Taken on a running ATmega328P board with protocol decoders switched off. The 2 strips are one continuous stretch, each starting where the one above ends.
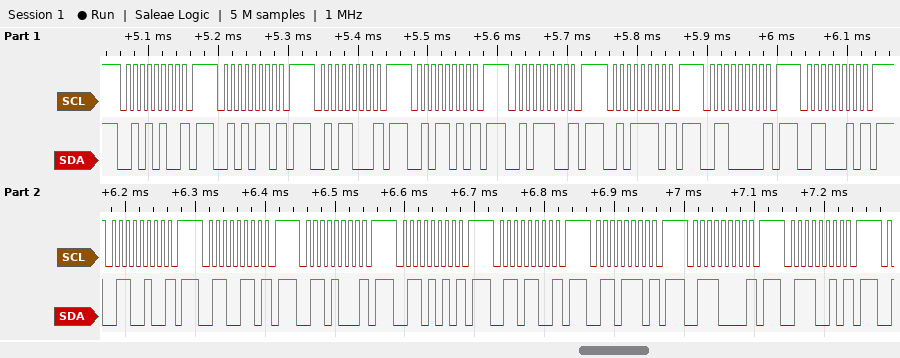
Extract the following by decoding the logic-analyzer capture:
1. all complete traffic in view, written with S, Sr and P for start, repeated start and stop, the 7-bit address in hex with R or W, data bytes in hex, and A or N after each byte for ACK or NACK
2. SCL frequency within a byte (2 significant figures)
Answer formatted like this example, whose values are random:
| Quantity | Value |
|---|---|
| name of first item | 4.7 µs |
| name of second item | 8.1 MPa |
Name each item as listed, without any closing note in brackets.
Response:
| Quantity | Value |
|---|---|
| all complete traffic in view, written with S, Sr and P for start, repeated start and stop, the 7-bit address in hex with R or W, data bytes in hex, and A or N after each byte for ACK or NACK | S 2AW N P S 2BW N P S 2CW N P S 2DW N P S 2EW N P S 2FW N P S 30W N P S 31W N P S 32W N P S 33W N P S 34W N P S 35W N P S 36W N P S 37W N P S 38W N P S 39W N P |
| SCL frequency within a byte | 100 kHz |
